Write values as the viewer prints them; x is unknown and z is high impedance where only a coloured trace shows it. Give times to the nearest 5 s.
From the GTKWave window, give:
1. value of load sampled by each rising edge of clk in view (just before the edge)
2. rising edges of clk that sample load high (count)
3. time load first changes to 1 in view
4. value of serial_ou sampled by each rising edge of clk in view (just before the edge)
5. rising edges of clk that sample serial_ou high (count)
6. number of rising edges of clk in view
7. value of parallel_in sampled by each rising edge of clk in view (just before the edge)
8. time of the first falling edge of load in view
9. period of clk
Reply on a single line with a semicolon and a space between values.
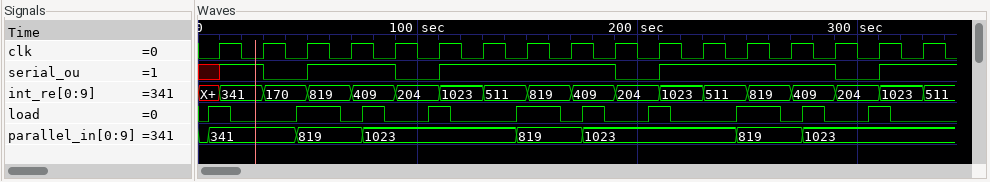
1 0 1 0 0 1 0 1 0 0 1 0 1 0 0 1 0; 7; 5 s; x 1 0 1 1 0 1 1 1 1 0 1 1 1 1 0 1; 12; 17; 341, 341, 819, 819, 1023, 1023, 1023, 819, 819, 1023, 1023, 1023, 819, 819, 1023, 1023, 1023; 15 s; 20 s
